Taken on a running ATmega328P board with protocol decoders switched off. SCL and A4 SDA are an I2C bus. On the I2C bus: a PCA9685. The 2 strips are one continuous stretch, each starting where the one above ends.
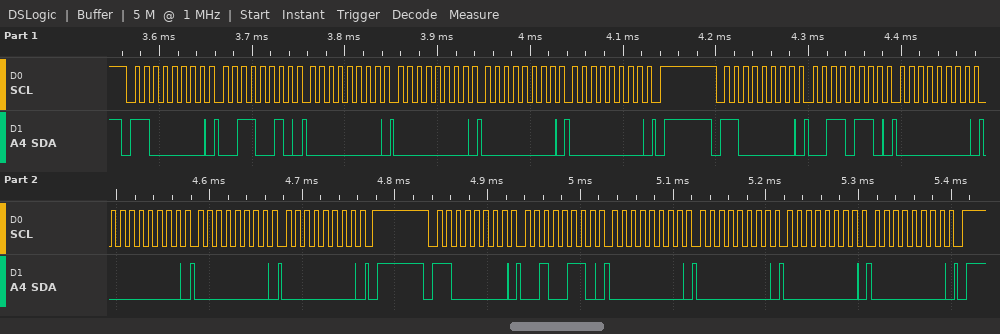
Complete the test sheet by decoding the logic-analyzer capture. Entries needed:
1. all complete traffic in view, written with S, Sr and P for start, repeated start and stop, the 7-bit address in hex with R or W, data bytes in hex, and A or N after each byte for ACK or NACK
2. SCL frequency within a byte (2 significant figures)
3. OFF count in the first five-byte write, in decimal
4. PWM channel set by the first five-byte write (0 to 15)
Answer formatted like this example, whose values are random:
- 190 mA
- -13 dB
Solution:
- S 60W A 32 A 00 A 00 A 00 A 00 A P S 60W A 36 A 00 A 00 A 00 A 00 A P S 60W A 26 A 00 A 00 A 00 A 00 A P
- 100 kHz
- 0
- 11
